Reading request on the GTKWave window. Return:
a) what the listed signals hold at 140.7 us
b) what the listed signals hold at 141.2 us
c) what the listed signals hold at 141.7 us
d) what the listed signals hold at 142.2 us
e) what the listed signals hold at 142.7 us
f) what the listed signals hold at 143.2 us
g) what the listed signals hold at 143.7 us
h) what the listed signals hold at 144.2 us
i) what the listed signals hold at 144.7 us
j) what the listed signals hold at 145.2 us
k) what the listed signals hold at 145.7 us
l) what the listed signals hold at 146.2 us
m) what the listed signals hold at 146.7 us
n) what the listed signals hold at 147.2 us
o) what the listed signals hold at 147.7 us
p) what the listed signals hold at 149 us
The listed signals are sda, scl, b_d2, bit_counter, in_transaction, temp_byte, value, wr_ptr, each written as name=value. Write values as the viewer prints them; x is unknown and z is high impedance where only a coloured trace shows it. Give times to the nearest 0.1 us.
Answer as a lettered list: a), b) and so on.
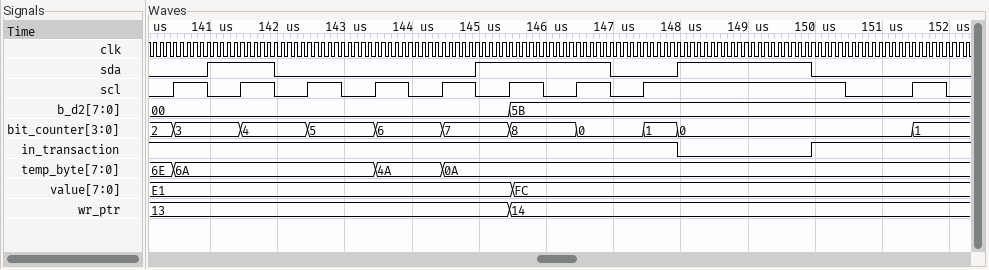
a) sda=0, scl=1, b_d2=00, bit_counter=3, in_transaction=1, temp_byte=6A, value=E1, wr_ptr=13
b) sda=1, scl=0, b_d2=00, bit_counter=3, in_transaction=1, temp_byte=6A, value=E1, wr_ptr=13
c) sda=1, scl=1, b_d2=00, bit_counter=4, in_transaction=1, temp_byte=6A, value=E1, wr_ptr=13
d) sda=0, scl=0, b_d2=00, bit_counter=4, in_transaction=1, temp_byte=6A, value=E1, wr_ptr=13
e) sda=0, scl=1, b_d2=00, bit_counter=5, in_transaction=1, temp_byte=6A, value=E1, wr_ptr=13
f) sda=0, scl=0, b_d2=00, bit_counter=5, in_transaction=1, temp_byte=6A, value=E1, wr_ptr=13
g) sda=0, scl=1, b_d2=00, bit_counter=6, in_transaction=1, temp_byte=4A, value=E1, wr_ptr=13
h) sda=0, scl=0, b_d2=00, bit_counter=6, in_transaction=1, temp_byte=4A, value=E1, wr_ptr=13
i) sda=0, scl=1, b_d2=00, bit_counter=7, in_transaction=1, temp_byte=0A, value=E1, wr_ptr=13
j) sda=1, scl=0, b_d2=00, bit_counter=7, in_transaction=1, temp_byte=0A, value=E1, wr_ptr=13
k) sda=1, scl=1, b_d2=5B, bit_counter=8, in_transaction=1, temp_byte=0A, value=FC, wr_ptr=14
l) sda=1, scl=0, b_d2=5B, bit_counter=8, in_transaction=1, temp_byte=0A, value=FC, wr_ptr=14
m) sda=1, scl=1, b_d2=5B, bit_counter=0, in_transaction=1, temp_byte=0A, value=FC, wr_ptr=14
n) sda=0, scl=0, b_d2=5B, bit_counter=0, in_transaction=1, temp_byte=0A, value=FC, wr_ptr=14
o) sda=0, scl=1, b_d2=5B, bit_counter=1, in_transaction=1, temp_byte=0A, value=FC, wr_ptr=14
p) sda=1, scl=1, b_d2=5B, bit_counter=0, in_transaction=0, temp_byte=0A, value=FC, wr_ptr=14
